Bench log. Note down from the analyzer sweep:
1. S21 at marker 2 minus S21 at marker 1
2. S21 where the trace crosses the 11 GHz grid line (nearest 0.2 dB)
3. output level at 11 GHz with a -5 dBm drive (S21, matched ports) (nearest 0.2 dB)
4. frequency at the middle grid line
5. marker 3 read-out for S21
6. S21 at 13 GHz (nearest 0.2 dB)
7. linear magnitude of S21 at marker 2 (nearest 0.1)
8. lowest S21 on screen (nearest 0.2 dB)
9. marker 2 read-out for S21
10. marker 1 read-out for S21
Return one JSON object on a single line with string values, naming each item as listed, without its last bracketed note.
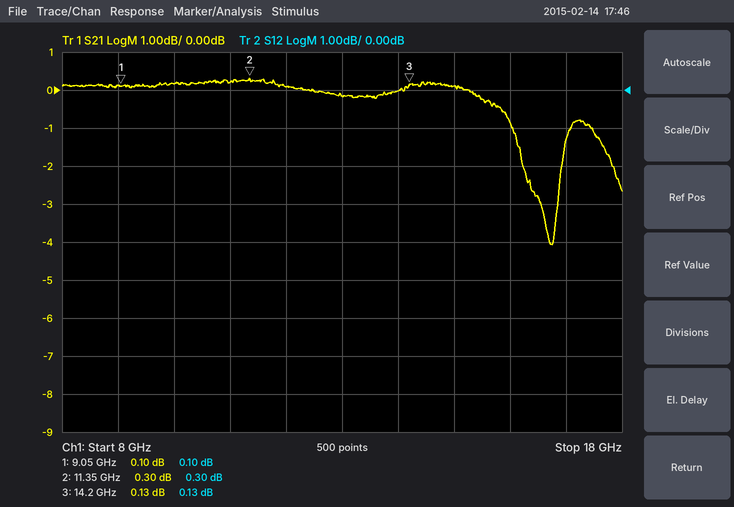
{"S21 at marker 2 minus S21 at marker 1": "0.20 dB", "S21 where the trace crosses the 11 GHz grid line": "0.2 dB", "output level at 11 GHz with a -5 dBm drive (S21, matched ports)": "-4.8 dBm", "frequency at the middle grid line": "13 GHz", "marker 3 read-out for S21": "0.13 dB", "S21 at 13 GHz": "-0.2 dB", "linear magnitude of S21 at marker 2": "1.0", "lowest S21 on screen": "-4.0 dB", "marker 2 read-out for S21": "0.30 dB", "marker 1 read-out for S21": "0.10 dB"}
